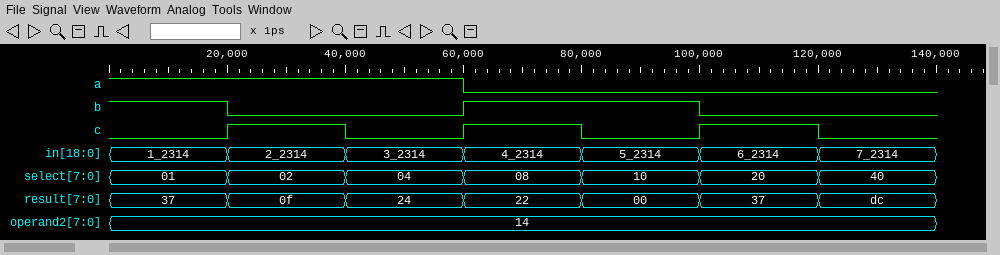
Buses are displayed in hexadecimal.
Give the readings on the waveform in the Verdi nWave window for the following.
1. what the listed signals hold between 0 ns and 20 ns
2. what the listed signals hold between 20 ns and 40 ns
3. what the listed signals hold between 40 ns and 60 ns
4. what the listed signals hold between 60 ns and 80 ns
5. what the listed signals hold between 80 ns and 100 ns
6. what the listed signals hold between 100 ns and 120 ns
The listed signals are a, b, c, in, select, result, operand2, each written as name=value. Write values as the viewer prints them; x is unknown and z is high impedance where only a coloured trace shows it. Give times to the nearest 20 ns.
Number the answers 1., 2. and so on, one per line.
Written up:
1. a=1, b=1, c=0, in=1_2314, select=01, result=37, operand2=14
2. a=1, b=0, c=1, in=2_2314, select=02, result=0f, operand2=14
3. a=1, b=0, c=0, in=3_2314, select=04, result=24, operand2=14
4. a=0, b=1, c=1, in=4_2314, select=08, result=22, operand2=14
5. a=0, b=1, c=0, in=5_2314, select=10, result=00, operand2=14
6. a=0, b=0, c=1, in=6_2314, select=20, result=37, operand2=14
